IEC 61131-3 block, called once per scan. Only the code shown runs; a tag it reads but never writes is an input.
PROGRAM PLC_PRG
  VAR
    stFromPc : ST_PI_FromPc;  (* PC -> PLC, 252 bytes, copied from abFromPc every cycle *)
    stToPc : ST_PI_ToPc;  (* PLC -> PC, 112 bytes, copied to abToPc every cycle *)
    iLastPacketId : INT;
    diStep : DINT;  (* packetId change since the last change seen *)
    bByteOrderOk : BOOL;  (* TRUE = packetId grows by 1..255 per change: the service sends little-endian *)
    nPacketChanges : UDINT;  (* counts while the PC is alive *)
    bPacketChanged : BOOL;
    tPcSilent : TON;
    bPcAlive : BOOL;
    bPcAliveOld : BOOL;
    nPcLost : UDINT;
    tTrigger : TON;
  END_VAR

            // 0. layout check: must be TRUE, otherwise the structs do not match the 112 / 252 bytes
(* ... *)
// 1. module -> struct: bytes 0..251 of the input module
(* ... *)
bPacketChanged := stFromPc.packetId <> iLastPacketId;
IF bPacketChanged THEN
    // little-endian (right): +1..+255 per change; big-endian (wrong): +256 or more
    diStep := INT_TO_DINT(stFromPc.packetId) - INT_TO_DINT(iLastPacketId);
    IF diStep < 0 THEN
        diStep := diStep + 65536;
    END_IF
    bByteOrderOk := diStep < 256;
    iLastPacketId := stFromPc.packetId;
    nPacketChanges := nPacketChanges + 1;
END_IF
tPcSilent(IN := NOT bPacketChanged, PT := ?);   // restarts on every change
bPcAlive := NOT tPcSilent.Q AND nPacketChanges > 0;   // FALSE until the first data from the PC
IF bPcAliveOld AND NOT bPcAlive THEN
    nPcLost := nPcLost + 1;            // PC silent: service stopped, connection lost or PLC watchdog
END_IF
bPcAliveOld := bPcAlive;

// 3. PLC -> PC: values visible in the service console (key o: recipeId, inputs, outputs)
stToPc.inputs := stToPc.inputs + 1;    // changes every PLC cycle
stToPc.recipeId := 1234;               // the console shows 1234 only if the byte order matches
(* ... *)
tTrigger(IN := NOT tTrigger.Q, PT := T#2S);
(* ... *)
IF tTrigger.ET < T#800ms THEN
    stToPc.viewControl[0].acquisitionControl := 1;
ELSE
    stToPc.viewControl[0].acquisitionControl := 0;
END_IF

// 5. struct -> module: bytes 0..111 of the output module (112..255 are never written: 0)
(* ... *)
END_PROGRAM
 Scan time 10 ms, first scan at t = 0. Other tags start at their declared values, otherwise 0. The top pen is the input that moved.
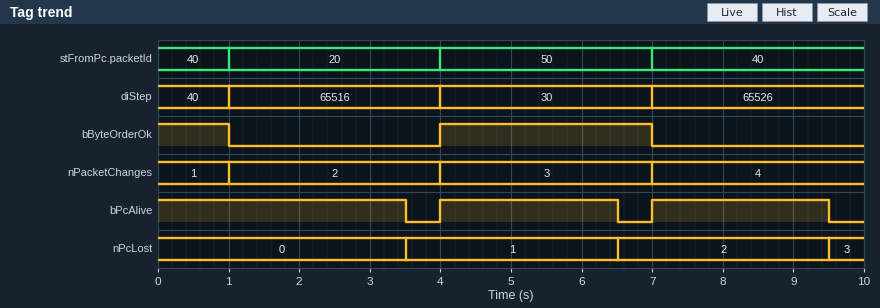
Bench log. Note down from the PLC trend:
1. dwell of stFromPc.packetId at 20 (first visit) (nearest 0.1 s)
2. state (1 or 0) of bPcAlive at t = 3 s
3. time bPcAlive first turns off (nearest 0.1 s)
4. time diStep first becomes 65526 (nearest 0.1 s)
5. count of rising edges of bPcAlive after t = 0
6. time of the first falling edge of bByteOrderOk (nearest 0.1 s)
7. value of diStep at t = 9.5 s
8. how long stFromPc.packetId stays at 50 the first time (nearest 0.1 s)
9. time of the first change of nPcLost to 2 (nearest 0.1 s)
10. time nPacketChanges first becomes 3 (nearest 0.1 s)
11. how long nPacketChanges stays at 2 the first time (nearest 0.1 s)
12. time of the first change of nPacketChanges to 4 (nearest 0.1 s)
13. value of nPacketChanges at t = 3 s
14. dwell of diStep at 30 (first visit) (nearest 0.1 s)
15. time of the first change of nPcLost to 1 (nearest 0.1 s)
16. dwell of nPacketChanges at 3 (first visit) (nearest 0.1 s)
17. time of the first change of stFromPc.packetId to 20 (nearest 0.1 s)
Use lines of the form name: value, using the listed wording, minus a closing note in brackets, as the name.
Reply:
dwell of stFromPc.packetId at 20 (first visit): 3.0 s
state (1 or 0) of bPcAlive at t = 3 s: 1
time bPcAlive first turns off: 3.5 s
time diStep first becomes 65526: 7.0 s
count of rising edges of bPcAlive after t = 0: 2
time of the first falling edge of bByteOrderOk: 1.0 s
value of diStep at t = 9.5 s: 65526
how long stFromPc.packetId stays at 50 the first time: 3.0 s
time of the first change of nPcLost to 2: 6.5 s
time nPacketChanges first becomes 3: 4.0 s
how long nPacketChanges stays at 2 the first time: 3.0 s
time of the first change of nPacketChanges to 4: 7.0 s
value of nPacketChanges at t = 3 s: 2
dwell of diStep at 30 (first visit): 3.0 s
time of the first change of nPcLost to 1: 3.5 s
dwell of nPacketChanges at 3 (first visit): 3.0 s
time of the first change of stFromPc.packetId to 20: 1.0 s
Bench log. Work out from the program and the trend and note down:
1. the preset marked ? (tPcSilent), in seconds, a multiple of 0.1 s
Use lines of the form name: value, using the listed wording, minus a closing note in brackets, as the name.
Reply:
the preset marked ? (tPcSilent), in seconds, a multiple of 0.1 s: 2.5 s
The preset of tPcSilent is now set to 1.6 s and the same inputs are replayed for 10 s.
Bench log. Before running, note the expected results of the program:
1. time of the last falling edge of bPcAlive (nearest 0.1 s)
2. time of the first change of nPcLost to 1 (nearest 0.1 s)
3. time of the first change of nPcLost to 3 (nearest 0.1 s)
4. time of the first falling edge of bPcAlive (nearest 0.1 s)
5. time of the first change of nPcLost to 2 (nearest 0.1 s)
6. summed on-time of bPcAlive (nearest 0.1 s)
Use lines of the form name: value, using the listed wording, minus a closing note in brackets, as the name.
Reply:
time of the last falling edge of bPcAlive: 8.6 s
time of the first change of nPcLost to 1: 2.6 s
time of the first change of nPcLost to 3: 8.6 s
time of the first falling edge of bPcAlive: 2.6 s
time of the first change of nPcLost to 2: 5.6 s
summed on-time of bPcAlive: 5.8 s
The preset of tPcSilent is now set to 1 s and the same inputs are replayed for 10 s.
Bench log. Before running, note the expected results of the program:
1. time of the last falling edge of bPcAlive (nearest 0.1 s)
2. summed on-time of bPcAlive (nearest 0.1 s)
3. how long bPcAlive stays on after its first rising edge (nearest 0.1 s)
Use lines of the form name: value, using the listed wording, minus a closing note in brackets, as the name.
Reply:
time of the last falling edge of bPcAlive: 8.0 s
summed on-time of bPcAlive: 4.0 s
how long bPcAlive stays on after its first rising edge: 1.0 s
